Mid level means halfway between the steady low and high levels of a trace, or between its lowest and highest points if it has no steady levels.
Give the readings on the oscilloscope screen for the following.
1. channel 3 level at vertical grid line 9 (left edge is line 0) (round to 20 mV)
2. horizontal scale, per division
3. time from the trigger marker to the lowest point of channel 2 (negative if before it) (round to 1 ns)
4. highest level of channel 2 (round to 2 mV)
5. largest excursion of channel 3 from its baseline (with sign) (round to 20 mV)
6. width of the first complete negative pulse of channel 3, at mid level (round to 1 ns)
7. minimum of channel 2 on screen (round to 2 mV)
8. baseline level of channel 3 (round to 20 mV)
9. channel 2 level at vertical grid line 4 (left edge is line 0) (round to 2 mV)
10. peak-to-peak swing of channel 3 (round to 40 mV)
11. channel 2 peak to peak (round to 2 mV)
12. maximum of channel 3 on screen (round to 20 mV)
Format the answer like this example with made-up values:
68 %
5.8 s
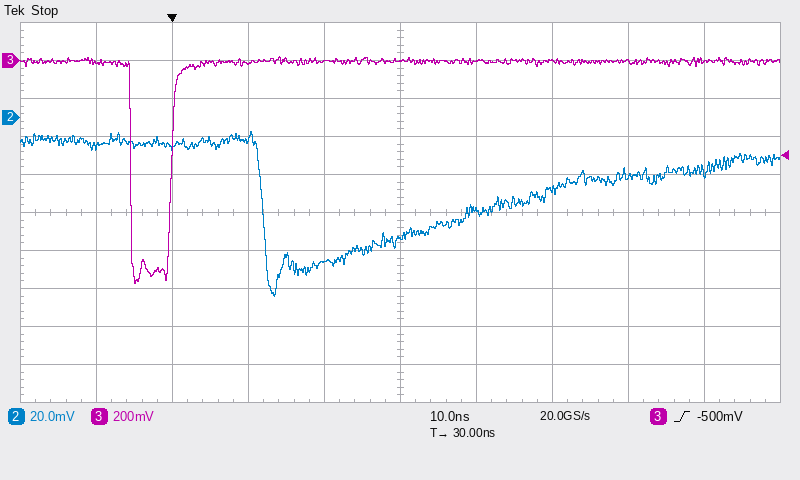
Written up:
0 mV
10 ns
+13 ns
-8 mV
-1.16 V
5 ns
-94 mV
0 mV
-76 mV
1.20 V
86 mV
20 mV
